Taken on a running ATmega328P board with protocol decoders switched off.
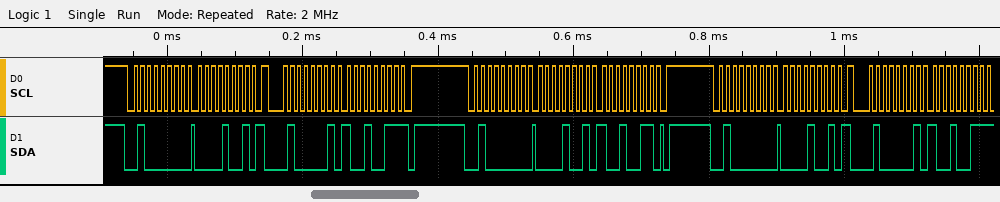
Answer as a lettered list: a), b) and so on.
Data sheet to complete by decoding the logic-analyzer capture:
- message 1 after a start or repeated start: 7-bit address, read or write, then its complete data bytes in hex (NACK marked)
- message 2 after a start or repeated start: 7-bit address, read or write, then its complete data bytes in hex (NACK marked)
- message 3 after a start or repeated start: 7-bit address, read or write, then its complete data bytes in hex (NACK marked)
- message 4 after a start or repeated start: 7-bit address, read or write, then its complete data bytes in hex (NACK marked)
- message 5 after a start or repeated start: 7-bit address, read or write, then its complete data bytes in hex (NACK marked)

a) 0x20 write: 09
b) 0x20 read: 93 NACK
c) 0x20 write: 09 93
d) 0x20 write: 09
e) 0x20 read: 93 NACK
